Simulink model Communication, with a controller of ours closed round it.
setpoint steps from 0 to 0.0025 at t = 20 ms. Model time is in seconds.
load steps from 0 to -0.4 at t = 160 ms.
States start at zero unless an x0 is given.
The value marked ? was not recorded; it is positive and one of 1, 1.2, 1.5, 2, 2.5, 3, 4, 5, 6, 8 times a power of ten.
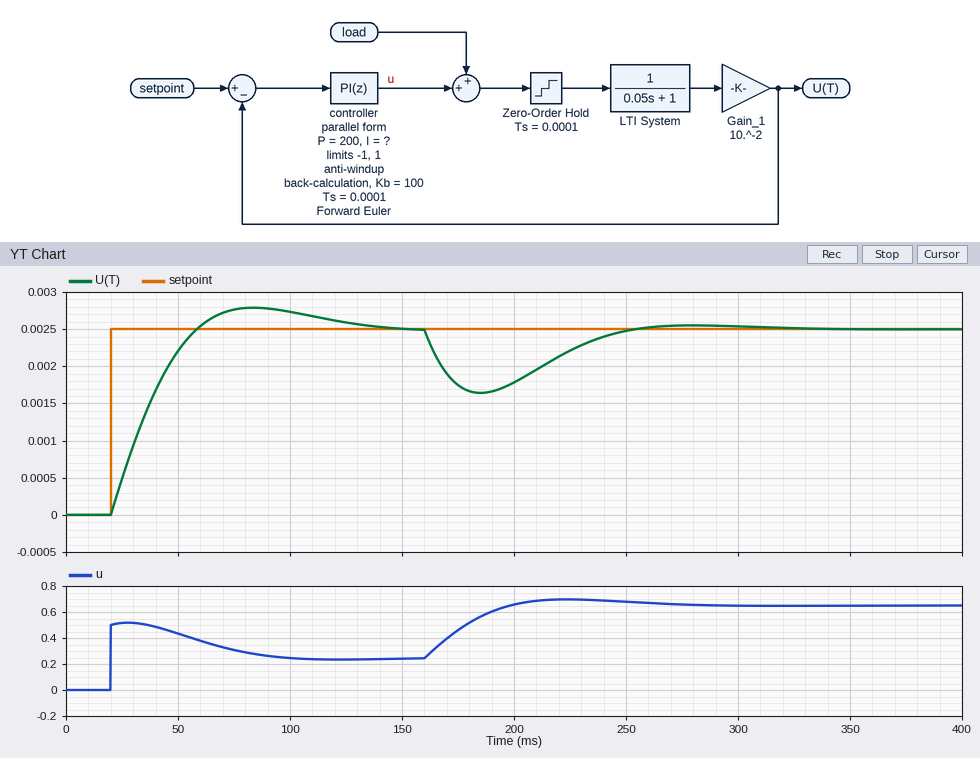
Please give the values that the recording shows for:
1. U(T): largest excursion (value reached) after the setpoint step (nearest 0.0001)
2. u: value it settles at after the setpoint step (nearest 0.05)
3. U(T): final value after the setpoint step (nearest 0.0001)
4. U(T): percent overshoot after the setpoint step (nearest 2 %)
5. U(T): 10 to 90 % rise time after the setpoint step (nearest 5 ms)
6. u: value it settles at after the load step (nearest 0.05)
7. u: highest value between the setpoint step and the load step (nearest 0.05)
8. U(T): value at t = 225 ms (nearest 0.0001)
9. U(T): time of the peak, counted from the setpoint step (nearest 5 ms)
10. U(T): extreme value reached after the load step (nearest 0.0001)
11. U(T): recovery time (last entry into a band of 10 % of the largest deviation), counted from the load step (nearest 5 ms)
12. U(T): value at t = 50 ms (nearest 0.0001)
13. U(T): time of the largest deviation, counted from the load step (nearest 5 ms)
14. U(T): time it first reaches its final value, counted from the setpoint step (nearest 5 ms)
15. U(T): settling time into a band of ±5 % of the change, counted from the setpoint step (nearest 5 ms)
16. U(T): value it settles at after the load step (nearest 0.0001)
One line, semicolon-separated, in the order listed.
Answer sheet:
0.0028; 0.25; 0.0025; 12 %; 30 ms; 0.65; 0.50; 0.0022; 65 ms; 0.0016; 80 ms; 0.0022; 25 ms; 40 ms; 100 ms; 0.0025
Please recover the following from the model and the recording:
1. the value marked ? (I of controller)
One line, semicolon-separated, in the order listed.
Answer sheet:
10000
